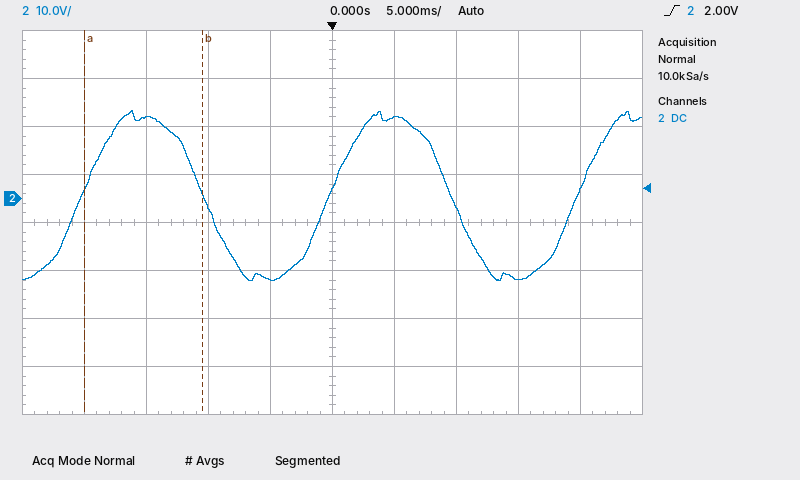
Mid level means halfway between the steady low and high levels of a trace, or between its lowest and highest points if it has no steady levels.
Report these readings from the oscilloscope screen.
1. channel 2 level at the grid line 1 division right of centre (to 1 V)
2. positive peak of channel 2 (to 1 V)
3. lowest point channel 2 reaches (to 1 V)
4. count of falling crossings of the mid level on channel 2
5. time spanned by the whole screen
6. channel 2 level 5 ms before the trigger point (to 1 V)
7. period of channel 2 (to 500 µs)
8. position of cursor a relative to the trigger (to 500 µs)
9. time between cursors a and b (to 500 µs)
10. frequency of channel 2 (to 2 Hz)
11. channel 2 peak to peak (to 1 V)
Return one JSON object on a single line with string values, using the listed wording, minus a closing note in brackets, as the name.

{"channel 2 level at the grid line 1 division right of centre": "17 V", "positive peak of channel 2": "18 V", "lowest point channel 2 reaches": "-17 V", "count of falling crossings of the mid level on channel 2": "2", "time spanned by the whole screen": "50 ms", "channel 2 level 5 ms before the trigger point": "-17 V", "period of channel 2": "20.0 ms", "position of cursor a relative to the trigger": "-20.0 ms", "time between cursors a and b": "9.5 ms", "frequency of channel 2": "50 Hz", "channel 2 peak to peak": "35 V"}
